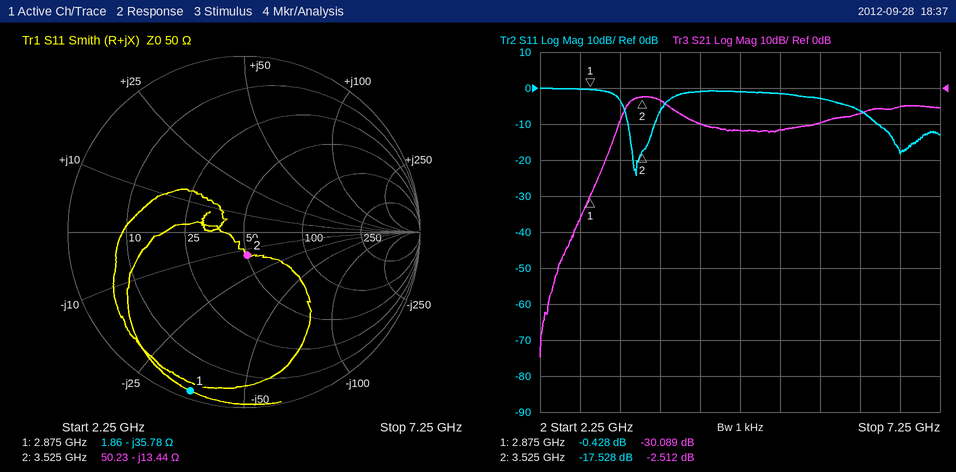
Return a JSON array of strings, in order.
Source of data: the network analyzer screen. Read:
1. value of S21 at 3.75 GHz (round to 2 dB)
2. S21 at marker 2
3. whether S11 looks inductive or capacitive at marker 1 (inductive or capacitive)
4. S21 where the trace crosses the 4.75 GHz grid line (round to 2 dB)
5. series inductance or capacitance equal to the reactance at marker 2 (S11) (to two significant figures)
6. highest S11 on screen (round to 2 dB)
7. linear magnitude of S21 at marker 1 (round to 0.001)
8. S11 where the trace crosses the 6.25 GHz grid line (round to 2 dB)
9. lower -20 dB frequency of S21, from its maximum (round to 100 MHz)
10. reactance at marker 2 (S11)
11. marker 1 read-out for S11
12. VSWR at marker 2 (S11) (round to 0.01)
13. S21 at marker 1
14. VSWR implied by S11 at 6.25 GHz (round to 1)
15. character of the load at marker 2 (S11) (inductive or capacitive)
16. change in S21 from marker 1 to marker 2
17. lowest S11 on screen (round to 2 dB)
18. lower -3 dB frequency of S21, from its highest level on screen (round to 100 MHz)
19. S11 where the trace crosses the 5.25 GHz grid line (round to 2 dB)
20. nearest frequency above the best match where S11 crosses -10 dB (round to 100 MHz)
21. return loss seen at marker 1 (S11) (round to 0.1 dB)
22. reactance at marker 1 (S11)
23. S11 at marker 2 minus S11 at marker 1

["-4 dB", "-2.512 dB", "capacitive", "-12 dB", "3.4 pF", "0 dB", "0.031", "-6 dB", "3.0 GHz", "-13.44 Ω", "-0.428 dB", "1.31", "-30.089 dB", "3", "capacitive", "27.577 dB", "-24 dB", "3.3 GHz", "-2 dB", "3.7 GHz", "0.4 dB", "-35.78 Ω", "-17.100 dB"]
